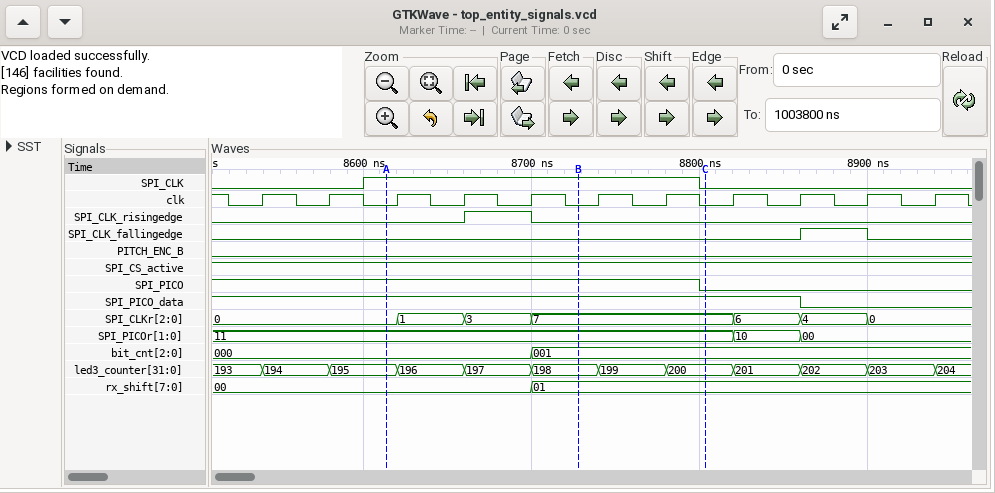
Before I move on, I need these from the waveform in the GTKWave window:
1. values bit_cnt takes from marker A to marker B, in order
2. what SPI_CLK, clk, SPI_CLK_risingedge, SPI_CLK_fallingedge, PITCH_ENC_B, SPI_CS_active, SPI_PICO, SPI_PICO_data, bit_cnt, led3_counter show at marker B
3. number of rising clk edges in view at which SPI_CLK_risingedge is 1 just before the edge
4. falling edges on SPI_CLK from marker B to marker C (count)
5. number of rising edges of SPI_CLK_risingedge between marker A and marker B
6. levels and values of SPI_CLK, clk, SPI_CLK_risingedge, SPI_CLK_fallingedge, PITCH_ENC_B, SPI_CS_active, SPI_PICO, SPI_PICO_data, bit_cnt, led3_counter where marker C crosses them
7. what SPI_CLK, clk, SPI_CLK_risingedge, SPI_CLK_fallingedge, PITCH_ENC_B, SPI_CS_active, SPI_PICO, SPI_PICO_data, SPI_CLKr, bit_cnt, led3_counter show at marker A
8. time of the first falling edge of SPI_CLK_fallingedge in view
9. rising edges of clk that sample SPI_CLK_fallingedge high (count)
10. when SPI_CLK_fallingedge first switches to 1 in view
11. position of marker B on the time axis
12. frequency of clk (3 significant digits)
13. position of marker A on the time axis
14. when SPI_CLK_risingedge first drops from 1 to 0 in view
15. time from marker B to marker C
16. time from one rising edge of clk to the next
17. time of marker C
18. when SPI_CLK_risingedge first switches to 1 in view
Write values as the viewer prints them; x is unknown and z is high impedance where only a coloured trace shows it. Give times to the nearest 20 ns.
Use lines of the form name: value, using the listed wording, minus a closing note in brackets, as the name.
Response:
values bit_cnt takes from marker A to marker B, in order: 000, 001
what SPI_CLK, clk, SPI_CLK_risingedge, SPI_CLK_fallingedge, PITCH_ENC_B, SPI_CS_active, SPI_PICO, SPI_PICO_data, bit_cnt, led3_counter show at marker B: SPI_CLK=1, clk=0, SPI_CLK_risingedge=0, SPI_CLK_fallingedge=0, PITCH_ENC_B=0, SPI_CS_active=1, SPI_PICO=1, SPI_PICO_data=1, bit_cnt=001, led3_counter=198
number of rising clk edges in view at which SPI_CLK_risingedge is 1 just before the edge: 1
falling edges on SPI_CLK from marker B to marker C: 1
number of rising edges of SPI_CLK_risingedge between marker A and marker B: 1
levels and values of SPI_CLK, clk, SPI_CLK_risingedge, SPI_CLK_fallingedge, PITCH_ENC_B, SPI_CS_active, SPI_PICO, SPI_PICO_data, bit_cnt, led3_counter where marker C crosses them: SPI_CLK=0, clk=0, SPI_CLK_risingedge=0, SPI_CLK_fallingedge=0, PITCH_ENC_B=0, SPI_CS_active=1, SPI_PICO=0, SPI_PICO_data=1, bit_cnt=001, led3_counter=200
what SPI_CLK, clk, SPI_CLK_risingedge, SPI_CLK_fallingedge, PITCH_ENC_B, SPI_CS_active, SPI_PICO, SPI_PICO_data, SPI_CLKr, bit_cnt, led3_counter show at marker A: SPI_CLK=1, clk=0, SPI_CLK_risingedge=0, SPI_CLK_fallingedge=0, PITCH_ENC_B=0, SPI_CS_active=1, SPI_PICO=1, SPI_PICO_data=1, SPI_CLKr=0, bit_cnt=000, led3_counter=195
time of the first falling edge of SPI_CLK_fallingedge in view: 8900 ns
rising edges of clk that sample SPI_CLK_fallingedge high: 1
when SPI_CLK_fallingedge first switches to 1 in view: 8860 ns
position of marker B on the time axis: 8720 ns
frequency of clk: 25.0 MHz
position of marker A on the time axis: 8620 ns
when SPI_CLK_risingedge first drops from 1 to 0 in view: 8700 ns
time from marker B to marker C: 80 ns
time from one rising edge of clk to the next: 40 ns
time of marker C: 8800 ns
when SPI_CLK_risingedge first switches to 1 in view: 8660 ns
